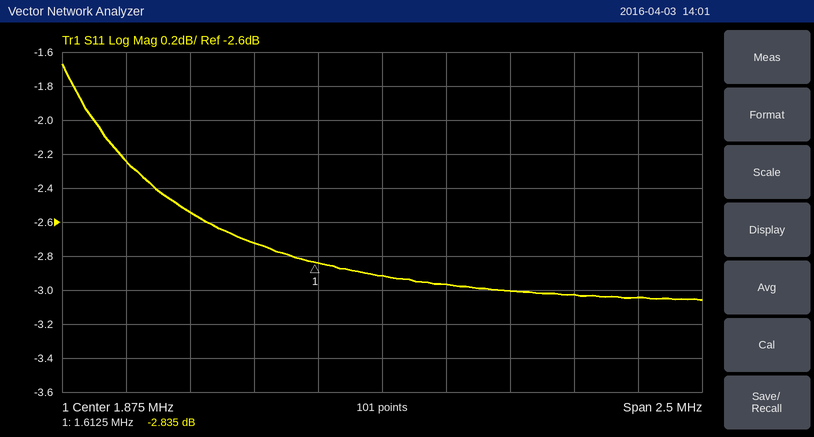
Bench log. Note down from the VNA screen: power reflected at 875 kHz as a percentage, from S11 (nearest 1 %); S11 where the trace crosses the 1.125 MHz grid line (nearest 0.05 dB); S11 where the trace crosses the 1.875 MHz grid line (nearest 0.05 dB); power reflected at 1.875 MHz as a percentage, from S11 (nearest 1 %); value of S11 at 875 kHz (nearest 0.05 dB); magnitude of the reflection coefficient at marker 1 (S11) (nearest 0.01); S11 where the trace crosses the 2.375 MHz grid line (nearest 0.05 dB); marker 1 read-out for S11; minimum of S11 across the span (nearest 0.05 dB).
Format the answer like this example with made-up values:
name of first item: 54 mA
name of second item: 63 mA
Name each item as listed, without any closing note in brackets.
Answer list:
power reflected at 875 kHz as a percentage, from S11: 60 %
S11 where the trace crosses the 1.125 MHz grid line: -2.55 dB
S11 where the trace crosses the 1.875 MHz grid line: -2.90 dB
power reflected at 1.875 MHz as a percentage, from S11: 51 %
value of S11 at 875 kHz: -2.25 dB
magnitude of the reflection coefficient at marker 1 (S11): 0.72
S11 where the trace crosses the 2.375 MHz grid line: -3.00 dB
marker 1 read-out for S11: -2.835 dB
minimum of S11 across the span: -3.05 dB
